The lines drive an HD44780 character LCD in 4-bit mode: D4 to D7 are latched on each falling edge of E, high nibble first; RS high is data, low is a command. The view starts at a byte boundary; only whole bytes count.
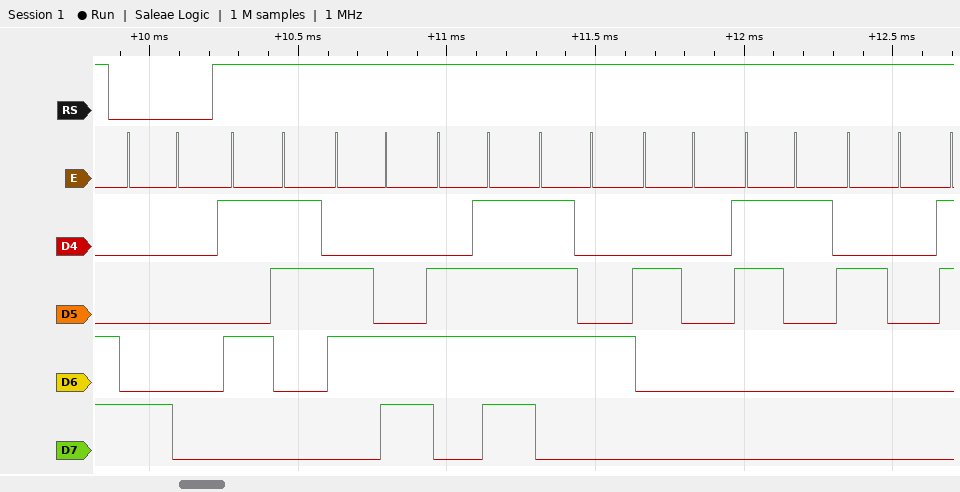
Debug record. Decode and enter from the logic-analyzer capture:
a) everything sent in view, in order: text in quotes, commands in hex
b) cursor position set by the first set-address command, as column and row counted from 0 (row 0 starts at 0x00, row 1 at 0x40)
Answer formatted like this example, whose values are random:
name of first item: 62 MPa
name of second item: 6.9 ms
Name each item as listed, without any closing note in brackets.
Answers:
everything sent in view, in order: text in quotes, commands in hex: 0x80 "Slot 1 "
cursor position set by the first set-address command, as column and row counted from 0: column 0, row 0
